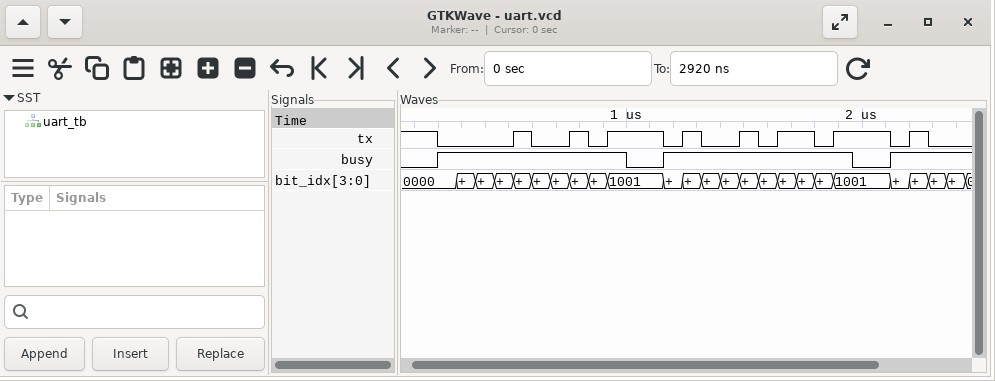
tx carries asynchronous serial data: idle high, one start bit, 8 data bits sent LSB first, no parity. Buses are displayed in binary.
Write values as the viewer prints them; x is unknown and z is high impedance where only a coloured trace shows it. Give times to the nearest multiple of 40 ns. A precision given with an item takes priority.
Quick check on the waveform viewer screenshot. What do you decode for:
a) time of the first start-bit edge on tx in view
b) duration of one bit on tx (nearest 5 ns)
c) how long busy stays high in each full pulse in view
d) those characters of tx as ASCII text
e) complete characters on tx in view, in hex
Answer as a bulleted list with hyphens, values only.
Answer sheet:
- 200 ns
- 80 ns
- 800 ns, 800 ns
- "Hi"
- 48, 69
